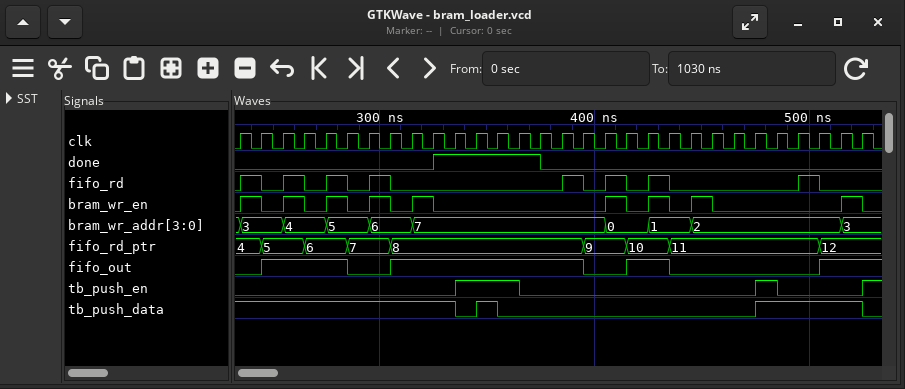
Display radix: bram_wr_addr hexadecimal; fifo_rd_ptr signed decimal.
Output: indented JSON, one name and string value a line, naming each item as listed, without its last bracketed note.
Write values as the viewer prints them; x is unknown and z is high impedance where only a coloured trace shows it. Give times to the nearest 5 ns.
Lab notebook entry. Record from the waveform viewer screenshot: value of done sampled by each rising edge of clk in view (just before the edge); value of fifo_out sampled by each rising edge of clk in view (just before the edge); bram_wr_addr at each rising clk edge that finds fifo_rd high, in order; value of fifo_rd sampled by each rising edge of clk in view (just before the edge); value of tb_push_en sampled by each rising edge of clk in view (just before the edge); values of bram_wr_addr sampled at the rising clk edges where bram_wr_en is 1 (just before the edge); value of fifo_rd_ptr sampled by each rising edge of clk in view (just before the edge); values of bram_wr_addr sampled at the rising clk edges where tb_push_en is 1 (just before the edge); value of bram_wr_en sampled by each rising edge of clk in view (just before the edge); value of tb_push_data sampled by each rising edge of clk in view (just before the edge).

{
  "value of done sampled by each rising edge of clk in view": "0 0 0 0 0 0 0 0 0 0 1 1 1 1 1 0 0 0 0 0 0 0 0 0 0 0 0 0 0 0",
  "value of fifo_out sampled by each rising edge of clk in view": "0 0 1 1 1 1 0 0 1 1 1 1 1 1 1 1 1 0 0 1 1 0 0 0 0 0 0 0 1 1",
  "bram_wr_addr at each rising clk edge that finds fifo_rd high, in order": "3, 4, 5, 6, 7, 0, 1, 2",
  "value of fifo_rd sampled by each rising edge of clk in view": "0 1 0 1 0 1 0 1 0 0 0 0 0 0 0 0 1 0 1 0 1 0 0 0 0 0 0 1 0 0",
  "value of tb_push_en sampled by each rising edge of clk in view": "0 0 0 0 0 0 0 0 0 0 0 1 1 1 0 0 0 0 0 0 0 0 0 0 0 1 0 0 0 0",
  "values of bram_wr_addr sampled at the rising clk edges where bram_wr_en is 1": "3, 4, 5, 6, 7, 0, 1, 2, 3",
  "value of fifo_rd_ptr sampled by each rising edge of clk in view": "4, 4, 5, 5, 6, 6, 7, 7, 8, 8, 8, 8, 8, 8, 8, 8, 8, 9, 9, 10, 10, 11, 11, 11, 11, 11, 11, 11, 12, 12",
  "values of bram_wr_addr sampled at the rising clk edges where tb_push_en is 1": "7, 7, 7, 2",
  "value of bram_wr_en sampled by each rising edge of clk in view": "0 1 0 1 0 1 0 1 0 1 0 0 0 0 0 0 0 0 1 0 1 0 1 0 0 0 0 0 0 1",
  "value of tb_push_data sampled by each rising edge of clk in view": "1 1 1 1 1 1 1 1 1 1 1 0 1 0 0 0 0 0 0 0 0 0 0 0 0 1 1 1 1 1"
}
